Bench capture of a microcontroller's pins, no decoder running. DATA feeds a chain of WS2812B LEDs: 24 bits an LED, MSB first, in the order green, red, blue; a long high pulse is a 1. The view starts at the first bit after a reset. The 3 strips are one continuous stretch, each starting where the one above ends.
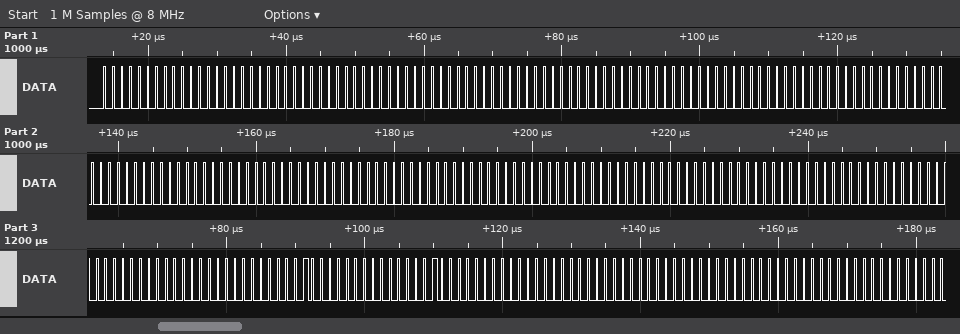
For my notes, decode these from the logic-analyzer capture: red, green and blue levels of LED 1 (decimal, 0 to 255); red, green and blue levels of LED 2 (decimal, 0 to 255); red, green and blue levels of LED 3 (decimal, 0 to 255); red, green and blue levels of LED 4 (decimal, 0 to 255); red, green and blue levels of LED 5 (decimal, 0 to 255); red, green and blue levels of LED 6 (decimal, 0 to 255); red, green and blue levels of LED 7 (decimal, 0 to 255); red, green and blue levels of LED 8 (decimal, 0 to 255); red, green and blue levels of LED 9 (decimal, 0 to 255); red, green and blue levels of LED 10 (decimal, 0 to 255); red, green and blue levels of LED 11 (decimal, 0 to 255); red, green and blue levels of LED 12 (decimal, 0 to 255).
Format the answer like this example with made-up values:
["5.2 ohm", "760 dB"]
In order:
["0, 0, 0", "0, 0, 0", "0, 0, 0", "0, 0, 0", "0, 0, 0", "0, 0, 0", "0, 0, 0", "0, 0, 0", "0, 0, 0", "0, 2, 4", "0, 0, 0", "0, 0, 0"]
